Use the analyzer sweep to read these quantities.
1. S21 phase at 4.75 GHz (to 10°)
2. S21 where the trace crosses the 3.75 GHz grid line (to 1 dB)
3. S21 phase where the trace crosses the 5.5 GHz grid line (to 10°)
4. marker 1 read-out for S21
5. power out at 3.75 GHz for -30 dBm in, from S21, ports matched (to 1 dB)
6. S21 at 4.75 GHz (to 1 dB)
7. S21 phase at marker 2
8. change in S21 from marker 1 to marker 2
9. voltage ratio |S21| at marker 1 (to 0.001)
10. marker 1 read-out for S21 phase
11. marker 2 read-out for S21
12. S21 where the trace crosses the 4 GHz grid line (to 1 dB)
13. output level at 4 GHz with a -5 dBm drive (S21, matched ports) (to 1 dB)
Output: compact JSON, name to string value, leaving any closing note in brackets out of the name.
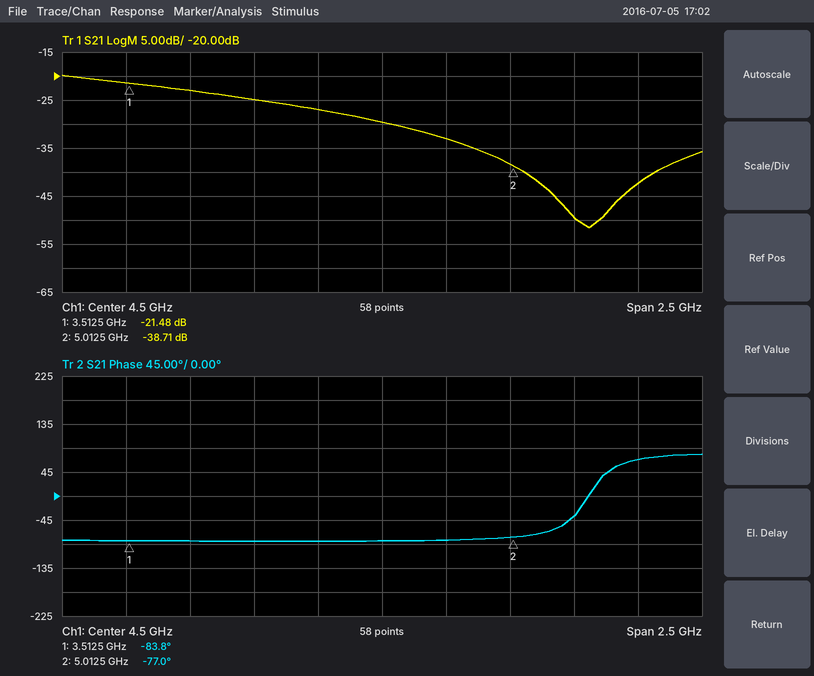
{"S21 phase at 4.75 GHz": "-80°", "S21 where the trace crosses the 3.75 GHz grid line": "-23 dB", "S21 phase where the trace crosses the 5.5 GHz grid line": "70°", "marker 1 read-out for S21": "-21.48 dB", "power out at 3.75 GHz for -30 dBm in, from S21, ports matched": "-53 dBm", "S21 at 4.75 GHz": "-33 dB", "S21 phase at marker 2": "-77.0°", "change in S21 from marker 1 to marker 2": "-17.23 dB", "voltage ratio |S21| at marker 1": "0.084", "marker 1 read-out for S21 phase": "-83.8°", "marker 2 read-out for S21": "-38.71 dB", "S21 where the trace crosses the 4 GHz grid line": "-25 dB", "output level at 4 GHz with a -5 dBm drive (S21, matched ports)": "-30 dBm"}
